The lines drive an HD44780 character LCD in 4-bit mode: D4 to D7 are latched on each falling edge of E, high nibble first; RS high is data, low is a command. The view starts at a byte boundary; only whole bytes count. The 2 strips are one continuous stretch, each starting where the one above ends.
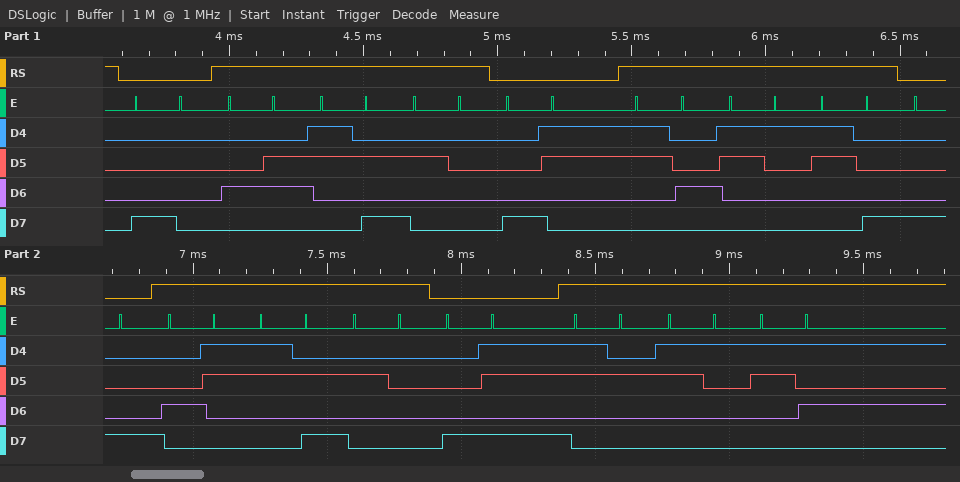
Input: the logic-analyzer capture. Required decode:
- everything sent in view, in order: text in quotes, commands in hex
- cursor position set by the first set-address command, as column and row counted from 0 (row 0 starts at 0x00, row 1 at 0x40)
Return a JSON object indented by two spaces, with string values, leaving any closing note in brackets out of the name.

{
  "everything sent in view, in order: text in quotes, commands in hex": "0x80 \"F: \" 0x83 \"418\" 0x88 \"C: \" 0x8B \"215\"",
  "cursor position set by the first set-address command, as column and row counted from 0": "column 0, row 0"
}
